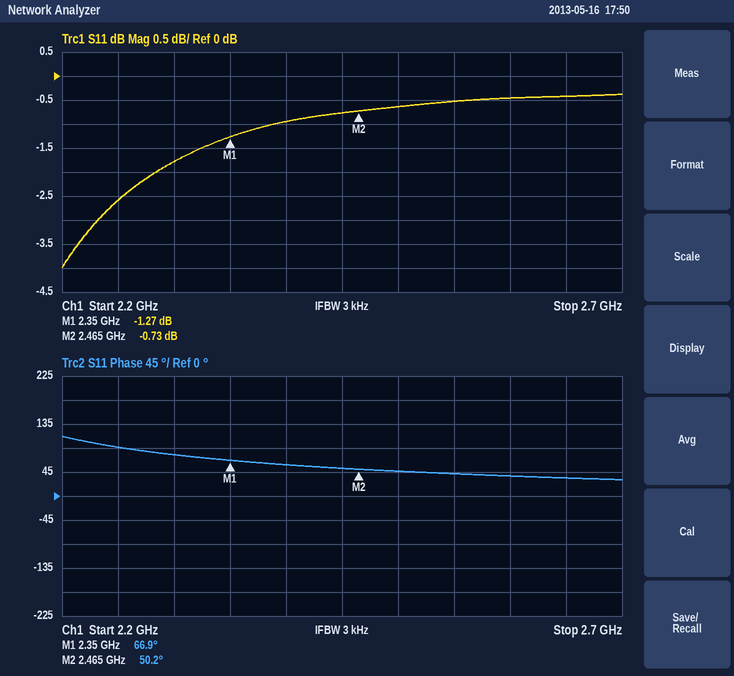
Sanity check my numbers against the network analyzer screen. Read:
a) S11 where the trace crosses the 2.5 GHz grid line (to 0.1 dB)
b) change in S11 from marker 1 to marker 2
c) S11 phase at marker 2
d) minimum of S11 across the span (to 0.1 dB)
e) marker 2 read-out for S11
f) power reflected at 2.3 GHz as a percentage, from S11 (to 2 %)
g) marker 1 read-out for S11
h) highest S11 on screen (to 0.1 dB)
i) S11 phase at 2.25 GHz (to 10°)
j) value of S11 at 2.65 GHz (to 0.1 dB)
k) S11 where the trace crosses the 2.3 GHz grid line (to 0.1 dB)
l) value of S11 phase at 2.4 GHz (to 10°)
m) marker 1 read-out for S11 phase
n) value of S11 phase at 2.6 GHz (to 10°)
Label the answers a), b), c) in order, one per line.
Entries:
a) -0.6 dB
b) 0.54 dB
c) 50.2°
d) -4.0 dB
e) -0.73 dB
f) 66 %
g) -1.27 dB
h) -0.4 dB
i) 90°
j) -0.4 dB
k) -1.8 dB
l) 60°
m) 66.9°
n) 40°
